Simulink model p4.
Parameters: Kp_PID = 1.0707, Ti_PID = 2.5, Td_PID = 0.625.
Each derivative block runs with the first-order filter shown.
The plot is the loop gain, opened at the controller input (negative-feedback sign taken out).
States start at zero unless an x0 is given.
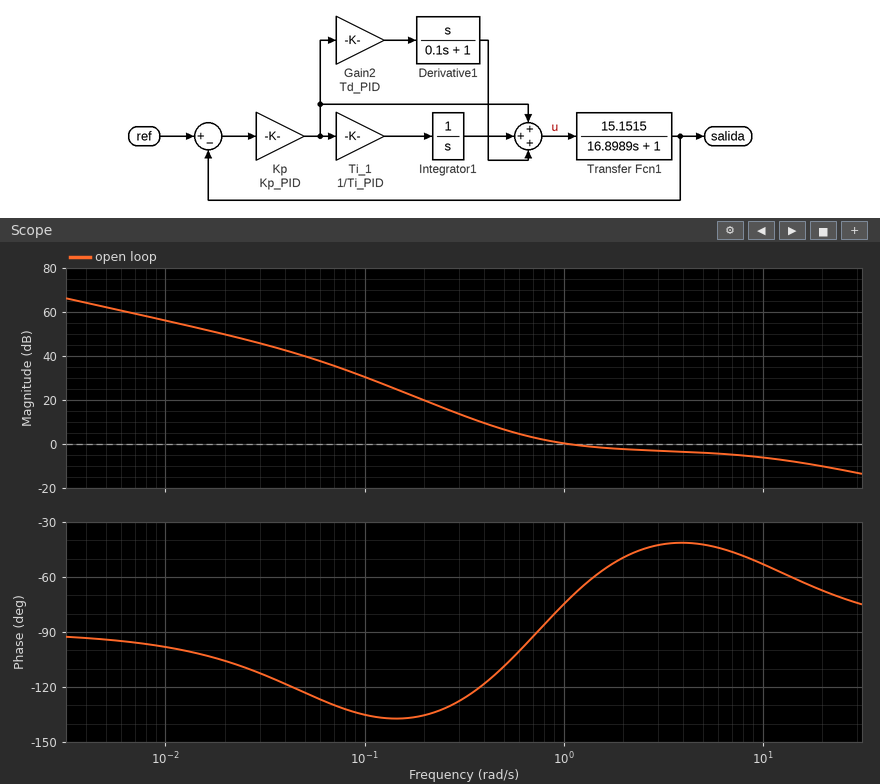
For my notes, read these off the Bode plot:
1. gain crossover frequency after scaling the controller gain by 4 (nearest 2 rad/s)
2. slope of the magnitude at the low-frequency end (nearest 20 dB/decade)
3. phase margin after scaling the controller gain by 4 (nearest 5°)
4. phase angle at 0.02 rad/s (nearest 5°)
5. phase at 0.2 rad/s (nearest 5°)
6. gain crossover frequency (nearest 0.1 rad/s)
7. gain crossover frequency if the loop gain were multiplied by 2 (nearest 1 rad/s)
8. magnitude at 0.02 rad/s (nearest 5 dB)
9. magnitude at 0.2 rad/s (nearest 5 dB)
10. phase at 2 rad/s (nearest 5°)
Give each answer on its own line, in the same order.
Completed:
26 rad/s
-20 dB/decade
110°
-105°
-135°
1.1 rad/s
10 rad/s
50 dB
20 dB
-50°
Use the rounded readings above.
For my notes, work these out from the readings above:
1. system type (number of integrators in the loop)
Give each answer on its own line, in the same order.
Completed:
1
